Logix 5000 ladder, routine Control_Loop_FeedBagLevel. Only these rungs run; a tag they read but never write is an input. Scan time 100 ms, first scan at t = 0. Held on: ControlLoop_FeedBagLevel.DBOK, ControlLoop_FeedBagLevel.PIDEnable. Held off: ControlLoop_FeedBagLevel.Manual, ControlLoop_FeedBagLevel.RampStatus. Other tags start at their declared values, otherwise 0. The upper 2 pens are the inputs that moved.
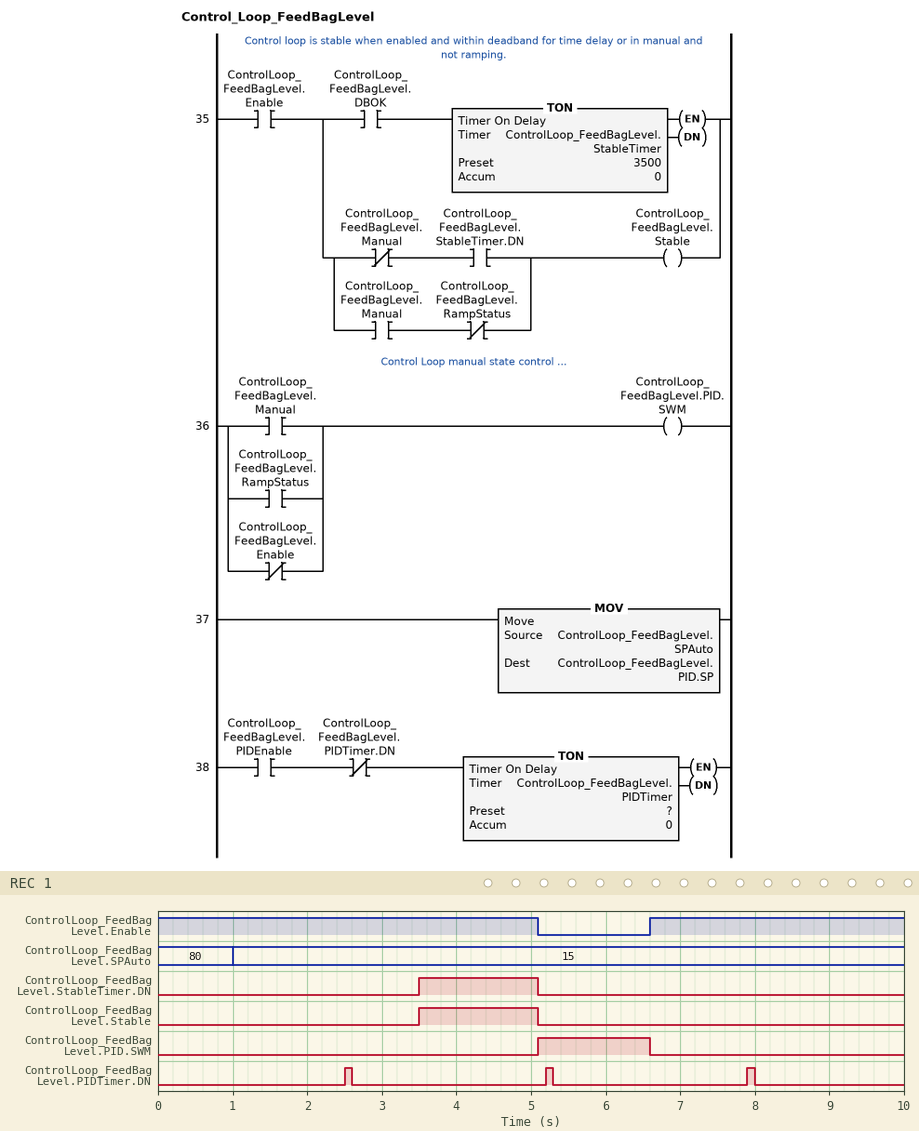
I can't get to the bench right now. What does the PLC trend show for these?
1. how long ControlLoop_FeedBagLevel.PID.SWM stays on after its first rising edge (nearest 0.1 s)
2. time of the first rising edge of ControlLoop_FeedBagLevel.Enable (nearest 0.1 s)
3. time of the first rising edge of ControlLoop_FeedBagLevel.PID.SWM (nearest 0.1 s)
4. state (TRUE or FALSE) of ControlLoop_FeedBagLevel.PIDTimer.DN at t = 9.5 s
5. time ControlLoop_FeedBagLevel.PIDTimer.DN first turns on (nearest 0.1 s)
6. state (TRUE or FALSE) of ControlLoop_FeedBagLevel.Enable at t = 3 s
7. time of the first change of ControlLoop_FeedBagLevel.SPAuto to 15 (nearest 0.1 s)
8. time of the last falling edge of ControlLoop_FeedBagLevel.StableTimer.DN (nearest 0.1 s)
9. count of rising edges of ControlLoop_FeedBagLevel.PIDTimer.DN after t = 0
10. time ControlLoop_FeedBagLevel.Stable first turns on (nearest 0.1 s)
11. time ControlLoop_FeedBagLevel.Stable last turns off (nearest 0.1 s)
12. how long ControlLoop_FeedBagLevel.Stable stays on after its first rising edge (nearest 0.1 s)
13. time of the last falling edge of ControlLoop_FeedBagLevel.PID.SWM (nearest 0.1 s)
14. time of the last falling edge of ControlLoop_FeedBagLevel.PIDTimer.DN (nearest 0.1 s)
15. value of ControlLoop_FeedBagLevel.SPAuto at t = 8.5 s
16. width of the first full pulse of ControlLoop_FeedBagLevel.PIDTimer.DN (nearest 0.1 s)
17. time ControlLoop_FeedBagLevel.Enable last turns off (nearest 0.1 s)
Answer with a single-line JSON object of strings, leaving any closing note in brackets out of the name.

{"how long ControlLoop_FeedBagLevel.PID.SWM stays on after its first rising edge": "1.5 s", "time of the first rising edge of ControlLoop_FeedBagLevel.Enable": "6.6 s", "time of the first rising edge of ControlLoop_FeedBagLevel.PID.SWM": "5.1 s", "state (TRUE or FALSE) of ControlLoop_FeedBagLevel.PIDTimer.DN at t = 9.5 s": "FALSE", "time ControlLoop_FeedBagLevel.PIDTimer.DN first turns on": "2.5 s", "state (TRUE or FALSE) of ControlLoop_FeedBagLevel.Enable at t = 3 s": "TRUE", "time of the first change of ControlLoop_FeedBagLevel.SPAuto to 15": "1.0 s", "time of the last falling edge of ControlLoop_FeedBagLevel.StableTimer.DN": "5.1 s", "count of rising edges of ControlLoop_FeedBagLevel.PIDTimer.DN after t = 0": "3", "time ControlLoop_FeedBagLevel.Stable first turns on": "3.5 s", "time ControlLoop_FeedBagLevel.Stable last turns off": "5.1 s", "how long ControlLoop_FeedBagLevel.Stable stays on after its first rising edge": "1.6 s", "time of the last falling edge of ControlLoop_FeedBagLevel.PID.SWM": "6.6 s", "time of the last falling edge of ControlLoop_FeedBagLevel.PIDTimer.DN": "8.0 s", "value of ControlLoop_FeedBagLevel.SPAuto at t = 8.5 s": "15", "width of the first full pulse of ControlLoop_FeedBagLevel.PIDTimer.DN": "0.1 s", "time ControlLoop_FeedBagLevel.Enable last turns off": "5.1 s"}
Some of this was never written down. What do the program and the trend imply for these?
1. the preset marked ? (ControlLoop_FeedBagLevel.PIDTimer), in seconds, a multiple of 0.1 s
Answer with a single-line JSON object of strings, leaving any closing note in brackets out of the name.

{"the preset marked ? (ControlLoop_FeedBagLevel.PIDTimer), in seconds, a multiple of 0.1 s": "2.5 s"}
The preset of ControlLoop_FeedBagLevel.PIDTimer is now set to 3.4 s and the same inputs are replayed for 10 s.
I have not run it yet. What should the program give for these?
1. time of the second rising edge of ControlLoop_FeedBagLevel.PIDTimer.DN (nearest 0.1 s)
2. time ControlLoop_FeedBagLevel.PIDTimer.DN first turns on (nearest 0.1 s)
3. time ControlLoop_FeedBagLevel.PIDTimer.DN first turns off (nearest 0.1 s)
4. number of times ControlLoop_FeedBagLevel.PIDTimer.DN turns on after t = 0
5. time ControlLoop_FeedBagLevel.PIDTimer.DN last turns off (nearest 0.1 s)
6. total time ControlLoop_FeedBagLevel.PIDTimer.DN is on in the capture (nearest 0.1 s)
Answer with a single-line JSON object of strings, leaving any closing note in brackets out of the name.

{"time of the second rising edge of ControlLoop_FeedBagLevel.PIDTimer.DN": "7.0 s", "time ControlLoop_FeedBagLevel.PIDTimer.DN first turns on": "3.4 s", "time ControlLoop_FeedBagLevel.PIDTimer.DN first turns off": "3.5 s", "number of times ControlLoop_FeedBagLevel.PIDTimer.DN turns on after t = 0": "2", "time ControlLoop_FeedBagLevel.PIDTimer.DN last turns off": "7.1 s", "total time ControlLoop_FeedBagLevel.PIDTimer.DN is on in the capture": "0.2 s"}
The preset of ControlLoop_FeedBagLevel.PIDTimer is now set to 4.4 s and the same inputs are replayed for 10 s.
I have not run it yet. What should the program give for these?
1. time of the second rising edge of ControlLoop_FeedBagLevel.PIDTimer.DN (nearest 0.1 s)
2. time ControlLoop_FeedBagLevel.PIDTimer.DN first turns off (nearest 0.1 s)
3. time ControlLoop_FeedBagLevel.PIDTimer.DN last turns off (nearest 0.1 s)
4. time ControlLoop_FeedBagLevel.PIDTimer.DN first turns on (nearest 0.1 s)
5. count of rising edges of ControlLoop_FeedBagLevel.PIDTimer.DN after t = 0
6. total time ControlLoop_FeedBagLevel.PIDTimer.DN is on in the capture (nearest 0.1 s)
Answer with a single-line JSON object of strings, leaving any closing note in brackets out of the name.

{"time of the second rising edge of ControlLoop_FeedBagLevel.PIDTimer.DN": "9.0 s", "time ControlLoop_FeedBagLevel.PIDTimer.DN first turns off": "4.5 s", "time ControlLoop_FeedBagLevel.PIDTimer.DN last turns off": "9.1 s", "time ControlLoop_FeedBagLevel.PIDTimer.DN first turns on": "4.4 s", "count of rising edges of ControlLoop_FeedBagLevel.PIDTimer.DN after t = 0": "2", "total time ControlLoop_FeedBagLevel.PIDTimer.DN is on in the capture": "0.2 s"}
